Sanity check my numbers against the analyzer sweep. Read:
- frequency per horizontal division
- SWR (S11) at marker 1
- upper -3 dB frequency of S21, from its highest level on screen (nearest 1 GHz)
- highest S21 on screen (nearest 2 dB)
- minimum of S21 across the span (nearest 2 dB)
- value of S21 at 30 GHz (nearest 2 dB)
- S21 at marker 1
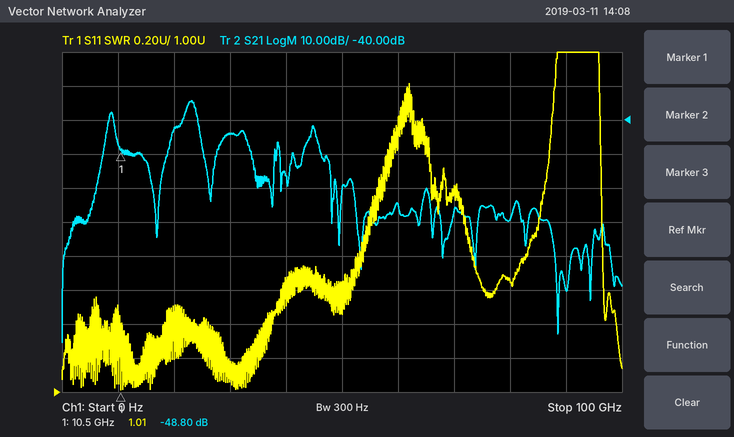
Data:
10 GHz
1.01
24 GHz
-34 dB
-106 dB
-44 dB
-48.80 dB
